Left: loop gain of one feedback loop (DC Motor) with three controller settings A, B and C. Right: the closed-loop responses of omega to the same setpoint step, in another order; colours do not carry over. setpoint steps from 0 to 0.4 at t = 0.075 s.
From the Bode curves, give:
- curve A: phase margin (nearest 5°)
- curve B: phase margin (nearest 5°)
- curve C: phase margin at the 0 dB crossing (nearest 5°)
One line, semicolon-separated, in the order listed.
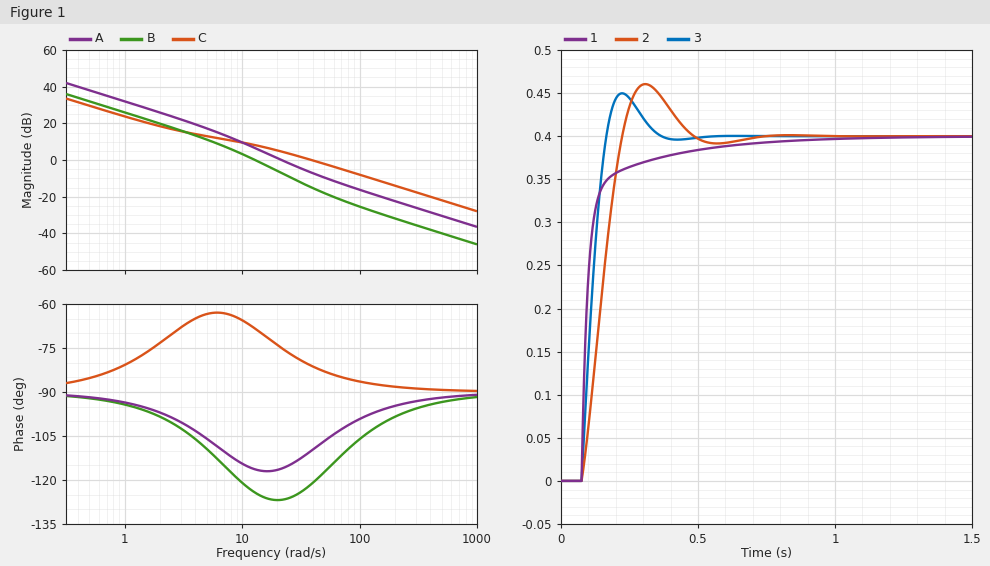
65°; 55°; 100°
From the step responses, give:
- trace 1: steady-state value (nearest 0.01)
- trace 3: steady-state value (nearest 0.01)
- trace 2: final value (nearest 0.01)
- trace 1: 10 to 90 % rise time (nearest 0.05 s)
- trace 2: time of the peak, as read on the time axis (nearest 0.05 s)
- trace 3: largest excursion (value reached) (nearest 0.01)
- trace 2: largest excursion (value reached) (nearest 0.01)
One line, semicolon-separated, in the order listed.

0.40; 0.40; 0.40; 0.15 s; 0.30 s; 0.45; 0.46
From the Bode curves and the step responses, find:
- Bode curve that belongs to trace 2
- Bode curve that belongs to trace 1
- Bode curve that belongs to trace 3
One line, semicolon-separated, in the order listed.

B; C; A
